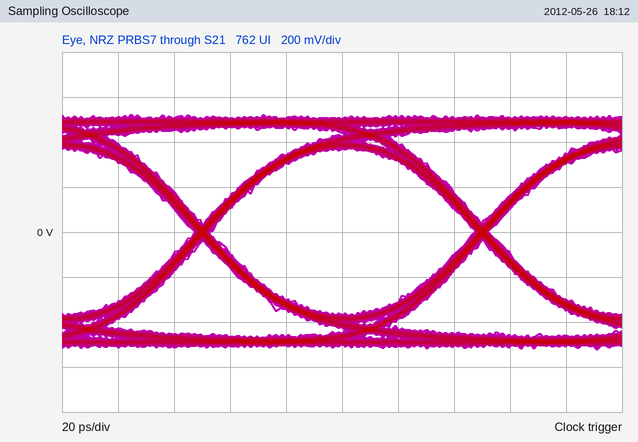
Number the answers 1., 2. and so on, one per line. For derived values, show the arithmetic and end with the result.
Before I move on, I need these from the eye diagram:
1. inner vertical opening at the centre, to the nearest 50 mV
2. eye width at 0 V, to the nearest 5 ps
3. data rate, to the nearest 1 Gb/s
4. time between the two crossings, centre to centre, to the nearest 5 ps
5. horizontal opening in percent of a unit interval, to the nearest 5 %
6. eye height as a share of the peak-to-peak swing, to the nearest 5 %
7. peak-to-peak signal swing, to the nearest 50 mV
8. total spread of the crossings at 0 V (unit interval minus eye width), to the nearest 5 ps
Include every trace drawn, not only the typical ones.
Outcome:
1. 750 mV
2. 95 ps
3. 10 Gb/s
4. 100 ps
5. 95 ps / 100 ps ≈ 95 %
6. 750 mV / 1.05 V ≈ 71.4 %, so 70 % to the nearest 5 %
7. 1.05 V
8. 5 ps
